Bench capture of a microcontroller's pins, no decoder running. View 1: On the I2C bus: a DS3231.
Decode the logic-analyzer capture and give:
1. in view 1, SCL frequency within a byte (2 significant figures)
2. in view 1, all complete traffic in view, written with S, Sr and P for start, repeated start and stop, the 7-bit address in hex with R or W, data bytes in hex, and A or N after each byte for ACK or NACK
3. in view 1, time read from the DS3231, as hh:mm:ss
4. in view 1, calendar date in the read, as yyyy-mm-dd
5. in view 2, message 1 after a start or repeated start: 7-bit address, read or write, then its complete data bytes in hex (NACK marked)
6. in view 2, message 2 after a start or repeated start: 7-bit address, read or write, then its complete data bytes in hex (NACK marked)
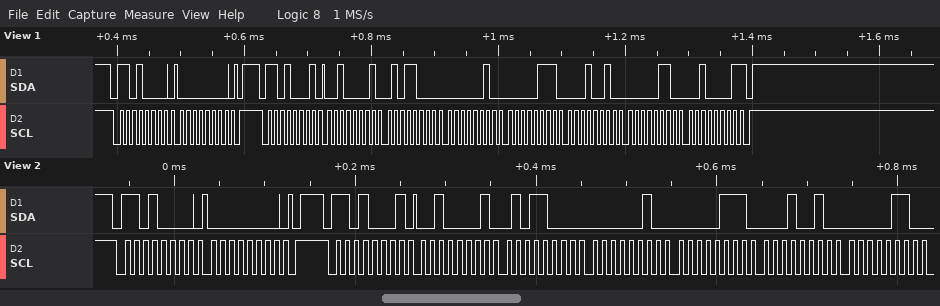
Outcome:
100 kHz
S 68W A 00 A P S 68R A 21 A 58 A 02 A 07 A 12 A 06 A 21 N P
02:58:21
2021-06-12
0x68 write: 00
0x68 read: 21 58 02 07 12 06
